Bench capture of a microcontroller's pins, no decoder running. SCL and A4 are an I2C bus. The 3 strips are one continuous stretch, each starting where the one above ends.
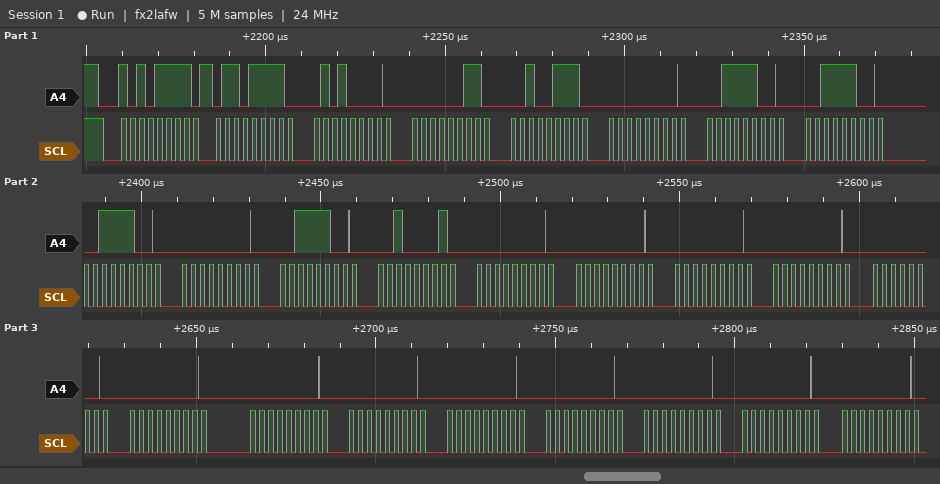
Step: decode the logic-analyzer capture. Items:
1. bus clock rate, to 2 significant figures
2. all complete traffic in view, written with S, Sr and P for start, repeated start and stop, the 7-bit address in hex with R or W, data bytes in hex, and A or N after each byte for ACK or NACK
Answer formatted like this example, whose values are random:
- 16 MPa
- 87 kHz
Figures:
- 400 kHz
- S 57R A 6F A 50 A 03 A 27 A 00 A 3C A 3C A 3C A 00 A 3C A 21 A 00 A 00 A 00 A 00 A 00 A 00 A 00 A 00 A 00 A 00 A 00 A 00 A 00 A
